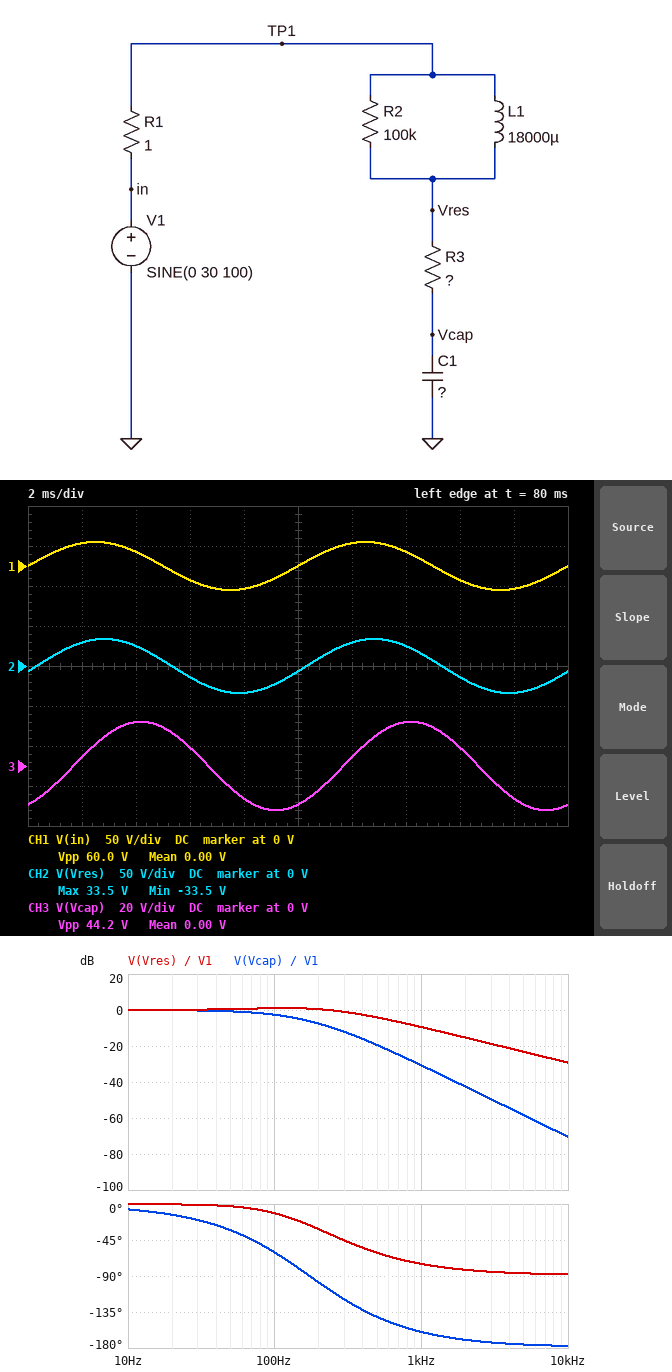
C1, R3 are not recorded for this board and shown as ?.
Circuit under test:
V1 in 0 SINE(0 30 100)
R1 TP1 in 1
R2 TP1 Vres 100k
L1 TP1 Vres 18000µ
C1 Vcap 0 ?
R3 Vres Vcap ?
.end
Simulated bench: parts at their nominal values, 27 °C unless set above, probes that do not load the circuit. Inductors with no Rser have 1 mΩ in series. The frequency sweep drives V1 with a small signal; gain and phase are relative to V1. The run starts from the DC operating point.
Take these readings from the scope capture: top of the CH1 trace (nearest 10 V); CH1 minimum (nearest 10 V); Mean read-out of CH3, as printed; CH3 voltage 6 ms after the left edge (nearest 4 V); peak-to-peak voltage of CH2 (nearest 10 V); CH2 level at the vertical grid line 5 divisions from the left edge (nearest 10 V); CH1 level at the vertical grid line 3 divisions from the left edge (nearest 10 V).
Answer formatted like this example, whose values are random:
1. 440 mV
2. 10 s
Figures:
1. 30 V
2. -30 V
3. 0.00 V
4. 8 V
5. 70 V
6. -10 V
7. -20 V
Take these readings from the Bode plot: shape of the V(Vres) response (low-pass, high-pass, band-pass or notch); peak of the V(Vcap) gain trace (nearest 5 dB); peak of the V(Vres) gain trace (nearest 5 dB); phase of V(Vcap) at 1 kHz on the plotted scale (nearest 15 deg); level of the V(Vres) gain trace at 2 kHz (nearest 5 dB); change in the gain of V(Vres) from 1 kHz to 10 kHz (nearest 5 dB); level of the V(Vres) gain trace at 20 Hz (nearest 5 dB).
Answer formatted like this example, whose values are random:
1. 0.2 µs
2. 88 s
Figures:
1. low-pass
2. 0 dB
3. 0 dB
4. -165 deg
5. -15 dB
6. -20 dB
7. 0 dB
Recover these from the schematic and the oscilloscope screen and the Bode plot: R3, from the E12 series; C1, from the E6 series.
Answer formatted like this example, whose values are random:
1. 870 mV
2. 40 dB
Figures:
1. 39 Ω
2. 47 µF
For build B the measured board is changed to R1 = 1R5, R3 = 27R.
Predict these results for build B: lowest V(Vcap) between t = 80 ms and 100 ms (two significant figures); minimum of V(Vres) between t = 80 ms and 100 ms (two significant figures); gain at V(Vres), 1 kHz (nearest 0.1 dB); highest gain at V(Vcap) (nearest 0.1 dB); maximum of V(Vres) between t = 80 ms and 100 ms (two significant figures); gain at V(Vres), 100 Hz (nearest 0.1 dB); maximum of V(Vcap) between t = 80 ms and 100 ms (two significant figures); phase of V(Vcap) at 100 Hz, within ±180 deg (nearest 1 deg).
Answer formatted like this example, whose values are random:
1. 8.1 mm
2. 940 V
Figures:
1. -28 V
2. -36 V
3. -12.4 dB
4. 0 dB
5. 36 V
6. 1.5 dB
7. 28 V
8. -52 deg
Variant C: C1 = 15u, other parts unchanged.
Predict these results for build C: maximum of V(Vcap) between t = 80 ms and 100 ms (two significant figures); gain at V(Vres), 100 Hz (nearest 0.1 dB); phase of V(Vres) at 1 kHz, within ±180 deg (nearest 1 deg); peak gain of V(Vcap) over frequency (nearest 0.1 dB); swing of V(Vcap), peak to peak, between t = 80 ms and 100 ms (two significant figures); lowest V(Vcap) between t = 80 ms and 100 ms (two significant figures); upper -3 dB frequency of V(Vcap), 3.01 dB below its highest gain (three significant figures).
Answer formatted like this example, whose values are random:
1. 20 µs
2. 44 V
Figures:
1. 31 V
2. 0.8 dB
3. -84 deg
4. 0.5 dB
5. 62 V
6. -31 V
7. 346 Hz
